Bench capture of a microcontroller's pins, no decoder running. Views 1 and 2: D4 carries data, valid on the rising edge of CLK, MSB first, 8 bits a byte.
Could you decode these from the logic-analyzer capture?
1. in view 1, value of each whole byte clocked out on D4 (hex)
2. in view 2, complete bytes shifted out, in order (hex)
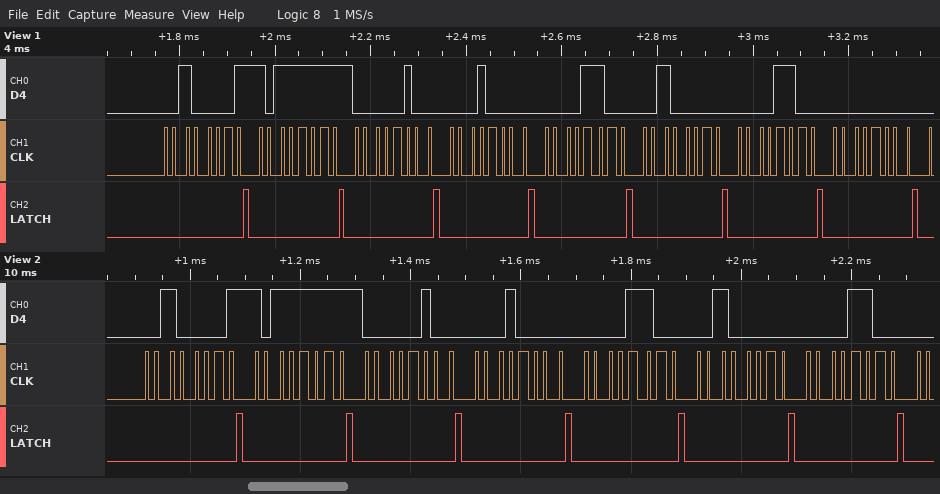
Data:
21 BF 04 10 0C 20 0C 00
21 BF 04 10 0C 20 0C
